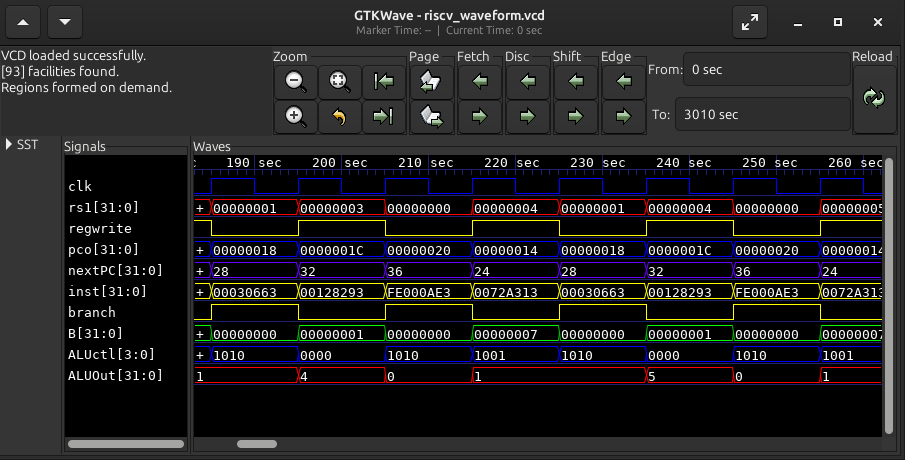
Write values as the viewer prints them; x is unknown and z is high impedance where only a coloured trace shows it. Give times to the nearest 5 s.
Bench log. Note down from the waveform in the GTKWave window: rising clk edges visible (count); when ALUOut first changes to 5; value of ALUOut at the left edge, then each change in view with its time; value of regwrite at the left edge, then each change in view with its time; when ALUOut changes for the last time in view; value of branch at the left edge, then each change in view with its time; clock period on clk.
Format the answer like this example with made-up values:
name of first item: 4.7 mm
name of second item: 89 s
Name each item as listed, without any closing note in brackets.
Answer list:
rising clk edges visible: 8
when ALUOut first changes to 5: 235 s
value of ALUOut at the left edge, then each change in view with its time: 1, 4 at 195 s, 0 at 205 s, 1 at 215 s, 5 at 235 s, 0 at 245 s, 1 at 255 s
value of regwrite at the left edge, then each change in view with its time: 1, 0 at 185 s, 1 at 195 s, 0 at 205 s, 1 at 215 s, 0 at 225 s, 1 at 235 s, 0 at 245 s, 1 at 255 s
when ALUOut changes for the last time in view: 255 s
value of branch at the left edge, then each change in view with its time: 0, 1 at 185 s, 0 at 195 s, 1 at 205 s, 0 at 215 s, 1 at 225 s, 0 at 235 s, 1 at 245 s, 0 at 255 s
clock period on clk: 10 s
